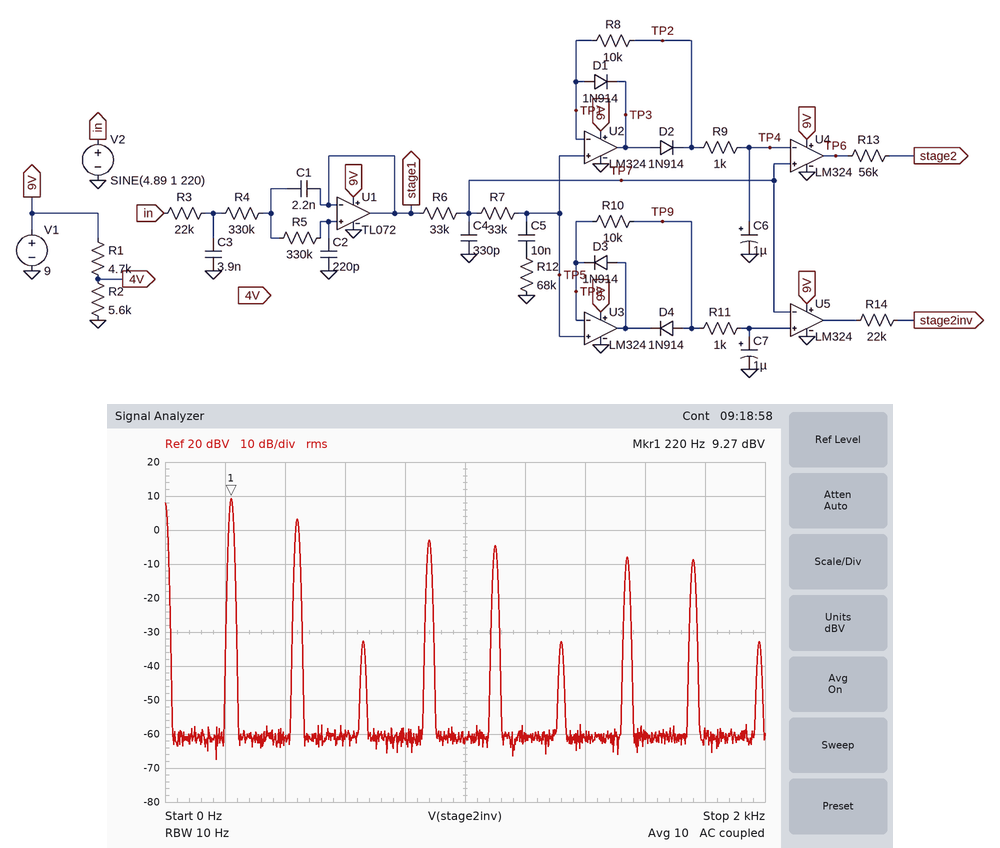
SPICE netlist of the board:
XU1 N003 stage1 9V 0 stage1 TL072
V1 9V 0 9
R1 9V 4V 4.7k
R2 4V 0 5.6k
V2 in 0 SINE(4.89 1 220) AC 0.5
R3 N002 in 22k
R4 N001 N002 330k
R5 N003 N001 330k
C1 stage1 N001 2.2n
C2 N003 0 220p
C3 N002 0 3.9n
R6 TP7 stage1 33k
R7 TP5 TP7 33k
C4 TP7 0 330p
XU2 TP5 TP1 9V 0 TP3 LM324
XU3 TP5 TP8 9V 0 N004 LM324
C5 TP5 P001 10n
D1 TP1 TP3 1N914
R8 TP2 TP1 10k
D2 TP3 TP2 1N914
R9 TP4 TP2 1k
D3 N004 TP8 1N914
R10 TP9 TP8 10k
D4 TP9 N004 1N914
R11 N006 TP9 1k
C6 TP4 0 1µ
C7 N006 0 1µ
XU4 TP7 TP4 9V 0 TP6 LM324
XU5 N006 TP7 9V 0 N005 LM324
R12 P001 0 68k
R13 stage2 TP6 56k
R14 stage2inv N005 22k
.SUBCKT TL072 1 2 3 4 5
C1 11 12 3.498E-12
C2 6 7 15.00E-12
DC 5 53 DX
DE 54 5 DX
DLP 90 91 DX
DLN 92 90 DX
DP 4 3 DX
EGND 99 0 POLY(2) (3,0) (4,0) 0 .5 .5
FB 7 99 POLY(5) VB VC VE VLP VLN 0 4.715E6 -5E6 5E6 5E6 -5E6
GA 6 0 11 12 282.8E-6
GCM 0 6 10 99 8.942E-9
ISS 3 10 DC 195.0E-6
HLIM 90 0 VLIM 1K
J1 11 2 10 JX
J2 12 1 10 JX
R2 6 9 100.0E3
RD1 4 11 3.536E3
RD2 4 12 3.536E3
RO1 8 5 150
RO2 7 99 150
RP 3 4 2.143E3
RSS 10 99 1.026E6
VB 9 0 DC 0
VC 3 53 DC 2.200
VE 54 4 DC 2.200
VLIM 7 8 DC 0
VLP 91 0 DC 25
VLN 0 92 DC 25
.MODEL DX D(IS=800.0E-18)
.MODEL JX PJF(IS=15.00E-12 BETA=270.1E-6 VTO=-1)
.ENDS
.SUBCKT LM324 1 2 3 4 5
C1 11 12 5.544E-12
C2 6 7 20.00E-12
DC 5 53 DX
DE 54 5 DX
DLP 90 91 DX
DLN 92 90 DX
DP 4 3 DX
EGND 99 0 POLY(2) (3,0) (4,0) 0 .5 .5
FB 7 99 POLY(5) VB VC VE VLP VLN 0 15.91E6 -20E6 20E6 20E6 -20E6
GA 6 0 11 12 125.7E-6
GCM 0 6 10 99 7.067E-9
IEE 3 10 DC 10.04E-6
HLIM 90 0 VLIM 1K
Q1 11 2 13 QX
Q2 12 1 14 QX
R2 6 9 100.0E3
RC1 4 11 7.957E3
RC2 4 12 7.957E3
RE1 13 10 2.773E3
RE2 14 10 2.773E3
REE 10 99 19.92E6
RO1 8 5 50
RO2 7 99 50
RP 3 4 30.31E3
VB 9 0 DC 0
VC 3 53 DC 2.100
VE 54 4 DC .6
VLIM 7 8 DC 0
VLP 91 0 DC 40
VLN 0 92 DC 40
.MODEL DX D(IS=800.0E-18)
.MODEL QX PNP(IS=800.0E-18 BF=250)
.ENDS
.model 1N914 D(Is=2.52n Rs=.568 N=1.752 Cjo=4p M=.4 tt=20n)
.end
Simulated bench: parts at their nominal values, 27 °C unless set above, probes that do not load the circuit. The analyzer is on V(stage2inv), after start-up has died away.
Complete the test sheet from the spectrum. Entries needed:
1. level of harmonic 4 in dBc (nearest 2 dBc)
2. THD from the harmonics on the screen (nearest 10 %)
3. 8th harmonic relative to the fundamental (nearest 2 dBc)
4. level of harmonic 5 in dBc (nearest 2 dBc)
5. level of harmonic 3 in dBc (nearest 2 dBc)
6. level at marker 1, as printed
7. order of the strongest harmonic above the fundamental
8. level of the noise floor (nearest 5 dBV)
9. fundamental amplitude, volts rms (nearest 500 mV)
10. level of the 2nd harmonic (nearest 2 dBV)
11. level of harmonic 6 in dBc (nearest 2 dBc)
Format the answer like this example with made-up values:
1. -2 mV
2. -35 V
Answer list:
1. -12 dBc
2. 60 %
3. -18 dBc
4. -14 dBc
5. -42 dBc
6. 9.27 dBV
7. 2
8. -60 dBV
9. 3.0 V
10. 4 dBV
11. -42 dBc
